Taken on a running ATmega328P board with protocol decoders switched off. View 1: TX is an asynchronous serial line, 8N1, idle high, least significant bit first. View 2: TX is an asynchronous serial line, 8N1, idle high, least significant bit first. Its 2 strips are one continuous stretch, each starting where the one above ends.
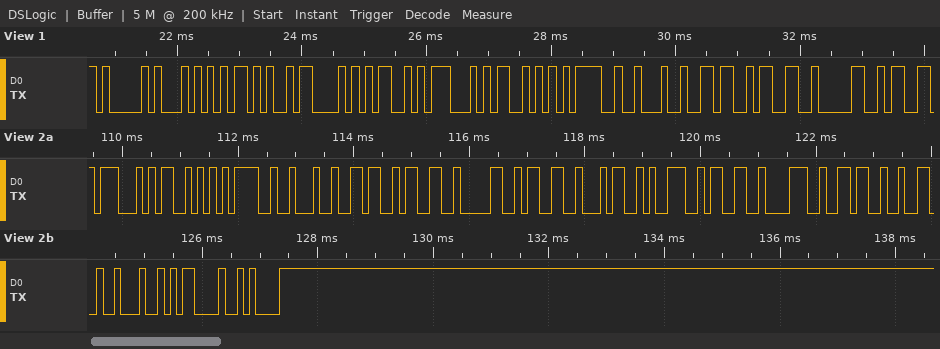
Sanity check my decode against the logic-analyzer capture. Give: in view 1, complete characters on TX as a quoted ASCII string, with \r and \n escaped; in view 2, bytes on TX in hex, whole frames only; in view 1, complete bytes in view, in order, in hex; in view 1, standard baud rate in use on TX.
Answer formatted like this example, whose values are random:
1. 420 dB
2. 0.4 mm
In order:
1. "AT+CMGS=\"630"
2. 47 53 3D 22 36 33 30 33 34 39 33 38 36 32 22 0D 0A
3. 41 54 2B 43 4D 47 53 3D 22 36 33 30
4. 9600 baud
